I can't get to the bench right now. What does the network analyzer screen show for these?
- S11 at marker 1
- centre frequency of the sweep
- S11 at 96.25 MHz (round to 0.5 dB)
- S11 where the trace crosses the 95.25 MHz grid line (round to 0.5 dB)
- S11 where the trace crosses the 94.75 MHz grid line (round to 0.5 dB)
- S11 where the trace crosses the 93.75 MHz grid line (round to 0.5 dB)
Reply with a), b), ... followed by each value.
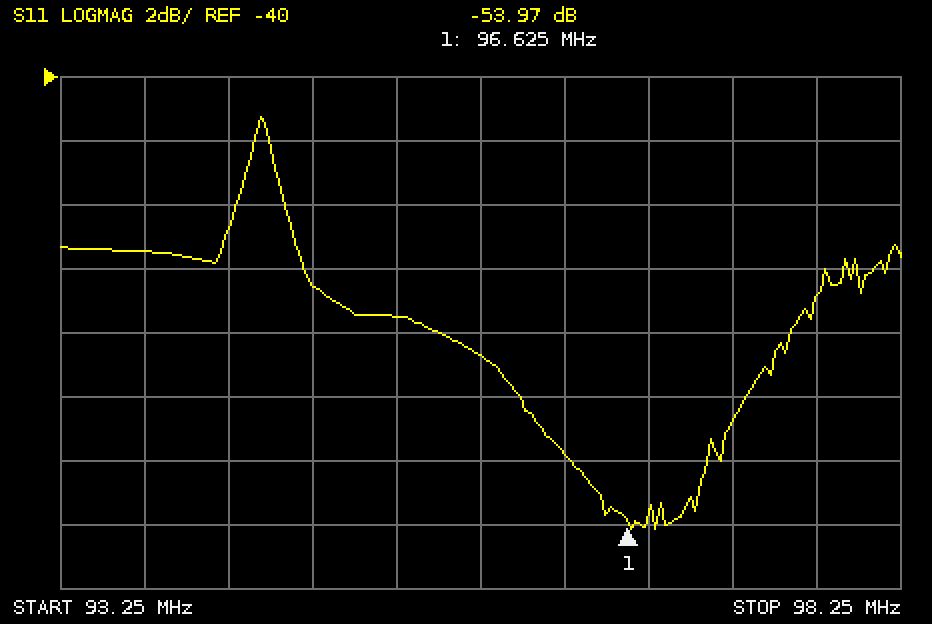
a) -53.97 dB
b) 95.75 MHz
c) -52.0 dB
d) -47.5 dB
e) -46.5 dB
f) -45.5 dB
